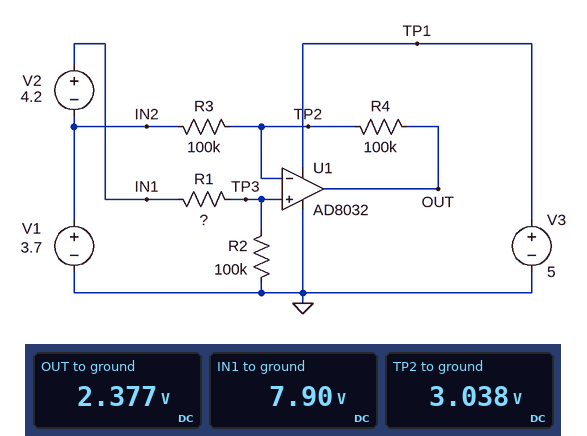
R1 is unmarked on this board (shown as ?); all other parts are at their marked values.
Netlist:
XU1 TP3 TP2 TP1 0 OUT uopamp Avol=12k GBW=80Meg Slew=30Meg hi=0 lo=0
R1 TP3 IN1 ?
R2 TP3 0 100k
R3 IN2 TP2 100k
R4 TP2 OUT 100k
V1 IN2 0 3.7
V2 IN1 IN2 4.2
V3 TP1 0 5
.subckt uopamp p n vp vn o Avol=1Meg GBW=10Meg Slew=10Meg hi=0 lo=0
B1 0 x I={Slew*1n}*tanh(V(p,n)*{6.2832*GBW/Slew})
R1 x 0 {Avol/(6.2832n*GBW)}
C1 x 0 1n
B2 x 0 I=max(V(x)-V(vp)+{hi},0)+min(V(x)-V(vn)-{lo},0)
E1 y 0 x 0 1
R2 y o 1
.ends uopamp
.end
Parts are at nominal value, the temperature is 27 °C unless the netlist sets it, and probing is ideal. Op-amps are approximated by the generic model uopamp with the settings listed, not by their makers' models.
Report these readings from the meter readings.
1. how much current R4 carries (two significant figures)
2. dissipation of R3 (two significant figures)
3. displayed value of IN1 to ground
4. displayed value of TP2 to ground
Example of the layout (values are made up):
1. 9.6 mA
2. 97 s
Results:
1. 6.6 µA
2. 4.4 µW
3. 7.90 V
4. 3.038 V
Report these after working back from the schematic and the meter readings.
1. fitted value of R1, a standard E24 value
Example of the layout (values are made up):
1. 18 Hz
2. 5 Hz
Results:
1. 160 kΩ
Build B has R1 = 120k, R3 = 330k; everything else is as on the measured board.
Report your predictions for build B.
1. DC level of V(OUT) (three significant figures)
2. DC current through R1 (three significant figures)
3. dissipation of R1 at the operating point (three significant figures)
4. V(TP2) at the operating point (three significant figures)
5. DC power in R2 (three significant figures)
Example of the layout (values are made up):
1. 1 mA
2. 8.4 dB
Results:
1. 3.56 V
2. 35.9 µA
3. 155 µW
4. 3.59 V
5. 129 µW
